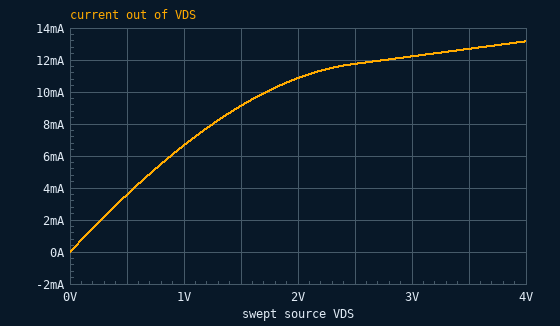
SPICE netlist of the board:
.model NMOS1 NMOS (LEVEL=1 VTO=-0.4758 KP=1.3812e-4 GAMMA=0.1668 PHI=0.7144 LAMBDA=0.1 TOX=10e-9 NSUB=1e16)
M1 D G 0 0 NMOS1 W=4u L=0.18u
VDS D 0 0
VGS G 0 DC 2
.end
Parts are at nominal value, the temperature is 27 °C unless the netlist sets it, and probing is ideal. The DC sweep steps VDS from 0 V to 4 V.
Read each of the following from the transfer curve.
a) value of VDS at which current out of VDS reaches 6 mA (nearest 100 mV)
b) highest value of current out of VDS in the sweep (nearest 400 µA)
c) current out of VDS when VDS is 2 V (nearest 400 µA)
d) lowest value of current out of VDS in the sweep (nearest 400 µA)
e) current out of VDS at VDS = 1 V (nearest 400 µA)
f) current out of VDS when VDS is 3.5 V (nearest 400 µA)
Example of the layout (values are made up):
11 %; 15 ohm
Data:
900 mV; 13.2 mA; 10.8 mA; 0 A; 6.8 mA; 12.8 mA
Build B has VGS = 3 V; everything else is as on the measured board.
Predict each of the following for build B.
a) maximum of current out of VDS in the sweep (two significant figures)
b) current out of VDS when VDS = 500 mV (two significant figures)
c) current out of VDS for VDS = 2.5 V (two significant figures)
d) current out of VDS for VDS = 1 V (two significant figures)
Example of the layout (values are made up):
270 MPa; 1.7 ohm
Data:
26 mA; 5.2 mA; 21 mA; 10 mA
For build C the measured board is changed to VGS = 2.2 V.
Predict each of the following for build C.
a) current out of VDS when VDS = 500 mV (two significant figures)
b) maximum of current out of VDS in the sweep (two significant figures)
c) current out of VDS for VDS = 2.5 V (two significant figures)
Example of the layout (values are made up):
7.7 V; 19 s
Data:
3.9 mA; 15 mA; 14 mA
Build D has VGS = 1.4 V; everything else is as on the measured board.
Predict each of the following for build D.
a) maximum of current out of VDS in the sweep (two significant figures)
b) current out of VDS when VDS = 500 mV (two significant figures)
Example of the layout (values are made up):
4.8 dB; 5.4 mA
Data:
7.6 mA; 2.6 mA
